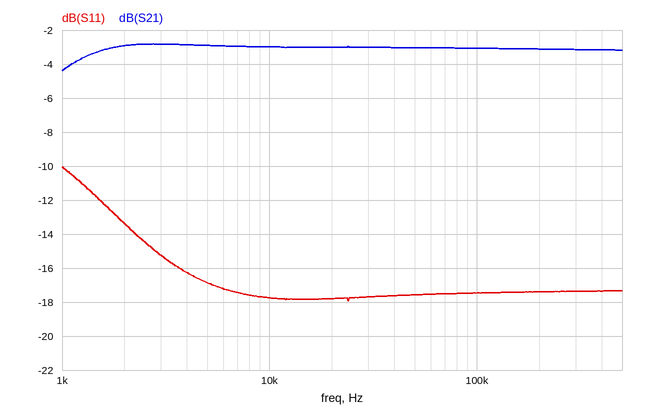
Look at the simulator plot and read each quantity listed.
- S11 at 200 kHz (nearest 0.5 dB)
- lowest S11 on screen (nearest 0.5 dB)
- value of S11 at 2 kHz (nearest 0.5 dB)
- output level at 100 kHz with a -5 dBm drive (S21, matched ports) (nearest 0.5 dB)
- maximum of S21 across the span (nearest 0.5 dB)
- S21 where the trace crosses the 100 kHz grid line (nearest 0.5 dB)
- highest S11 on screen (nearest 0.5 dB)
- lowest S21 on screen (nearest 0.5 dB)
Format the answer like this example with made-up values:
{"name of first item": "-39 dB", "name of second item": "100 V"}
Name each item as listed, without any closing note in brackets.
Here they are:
{"S11 at 200 kHz": "-17.5 dB", "lowest S11 on screen": "-18.0 dB", "value of S11 at 2 kHz": "-13.5 dB", "output level at 100 kHz with a -5 dBm drive (S21, matched ports)": "-8.0 dBm", "maximum of S21 across the span": "-3.0 dB", "S21 where the trace crosses the 100 kHz grid line": "-3.0 dB", "highest S11 on screen": "-10.0 dB", "lowest S21 on screen": "-4.5 dB"}
